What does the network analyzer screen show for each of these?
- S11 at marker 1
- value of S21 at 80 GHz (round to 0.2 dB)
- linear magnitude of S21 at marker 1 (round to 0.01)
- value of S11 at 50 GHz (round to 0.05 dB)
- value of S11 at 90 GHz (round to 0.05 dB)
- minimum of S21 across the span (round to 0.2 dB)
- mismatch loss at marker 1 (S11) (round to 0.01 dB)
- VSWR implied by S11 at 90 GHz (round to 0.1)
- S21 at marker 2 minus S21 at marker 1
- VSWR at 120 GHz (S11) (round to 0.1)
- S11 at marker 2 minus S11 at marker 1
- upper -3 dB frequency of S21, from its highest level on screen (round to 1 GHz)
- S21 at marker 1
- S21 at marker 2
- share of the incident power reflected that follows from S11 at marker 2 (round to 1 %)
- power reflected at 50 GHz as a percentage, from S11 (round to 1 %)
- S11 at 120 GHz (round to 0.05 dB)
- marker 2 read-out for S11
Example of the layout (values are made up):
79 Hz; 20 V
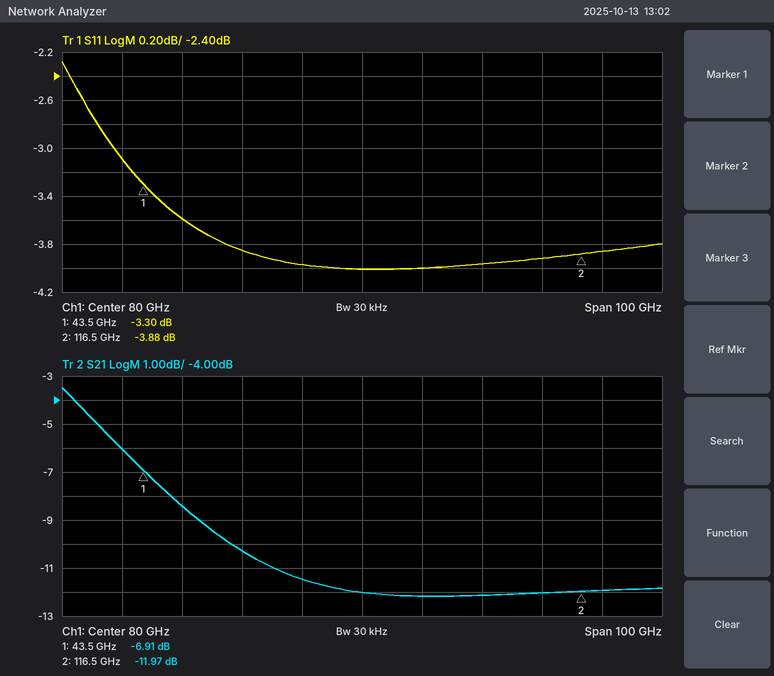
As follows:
-3.30 dB; -12.0 dB; 0.45; -3.60 dB; -4.00 dB; -12.2 dB; 2.74 dB; 4.4; -5.06 dB; 4.6; -0.58 dB; 42 GHz; -6.91 dB; -11.97 dB; 41 %; 44 %; -3.85 dB; -3.88 dB
